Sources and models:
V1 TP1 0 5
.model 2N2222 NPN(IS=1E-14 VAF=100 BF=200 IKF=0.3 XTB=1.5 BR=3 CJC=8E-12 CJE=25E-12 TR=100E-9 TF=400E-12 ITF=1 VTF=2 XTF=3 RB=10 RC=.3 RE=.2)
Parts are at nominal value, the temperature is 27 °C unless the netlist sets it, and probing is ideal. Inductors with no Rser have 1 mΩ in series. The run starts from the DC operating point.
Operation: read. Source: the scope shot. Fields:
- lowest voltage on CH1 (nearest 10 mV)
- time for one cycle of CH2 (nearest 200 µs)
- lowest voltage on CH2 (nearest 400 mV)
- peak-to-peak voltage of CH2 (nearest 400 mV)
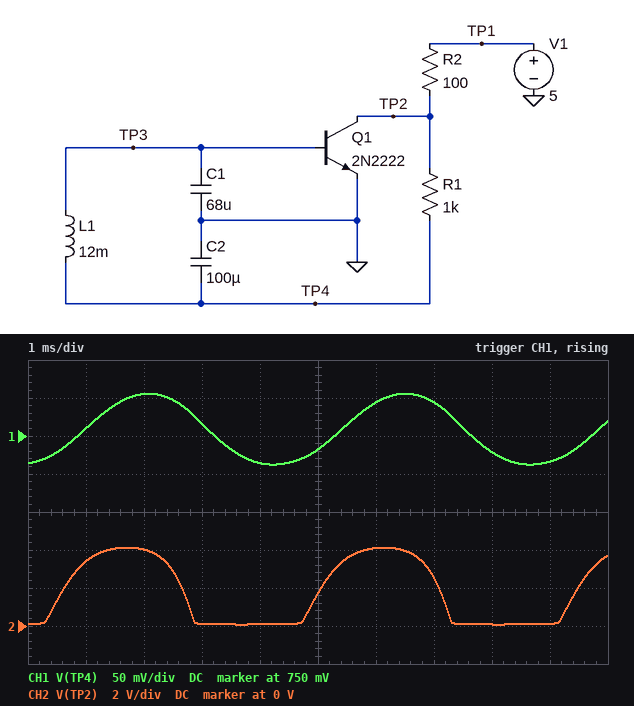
710 mV
4.4 ms
0 V
4.0 V
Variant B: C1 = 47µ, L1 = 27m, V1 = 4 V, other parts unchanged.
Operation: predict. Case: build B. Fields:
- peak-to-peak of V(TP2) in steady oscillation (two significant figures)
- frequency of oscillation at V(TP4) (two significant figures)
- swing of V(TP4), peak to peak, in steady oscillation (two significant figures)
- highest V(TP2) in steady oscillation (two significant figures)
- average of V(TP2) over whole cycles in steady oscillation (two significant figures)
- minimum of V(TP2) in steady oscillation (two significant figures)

3.0 V
170 Hz
61 mV
3.1 V
1.3 V
81 mV
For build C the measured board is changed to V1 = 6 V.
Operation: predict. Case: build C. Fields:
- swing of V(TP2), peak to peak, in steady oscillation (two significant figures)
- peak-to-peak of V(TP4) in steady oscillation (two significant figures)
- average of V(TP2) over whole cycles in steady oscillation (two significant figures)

4.8 V
100 mV
2.0 V
